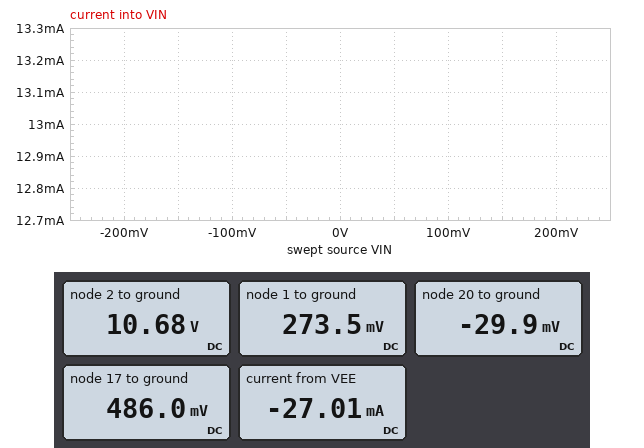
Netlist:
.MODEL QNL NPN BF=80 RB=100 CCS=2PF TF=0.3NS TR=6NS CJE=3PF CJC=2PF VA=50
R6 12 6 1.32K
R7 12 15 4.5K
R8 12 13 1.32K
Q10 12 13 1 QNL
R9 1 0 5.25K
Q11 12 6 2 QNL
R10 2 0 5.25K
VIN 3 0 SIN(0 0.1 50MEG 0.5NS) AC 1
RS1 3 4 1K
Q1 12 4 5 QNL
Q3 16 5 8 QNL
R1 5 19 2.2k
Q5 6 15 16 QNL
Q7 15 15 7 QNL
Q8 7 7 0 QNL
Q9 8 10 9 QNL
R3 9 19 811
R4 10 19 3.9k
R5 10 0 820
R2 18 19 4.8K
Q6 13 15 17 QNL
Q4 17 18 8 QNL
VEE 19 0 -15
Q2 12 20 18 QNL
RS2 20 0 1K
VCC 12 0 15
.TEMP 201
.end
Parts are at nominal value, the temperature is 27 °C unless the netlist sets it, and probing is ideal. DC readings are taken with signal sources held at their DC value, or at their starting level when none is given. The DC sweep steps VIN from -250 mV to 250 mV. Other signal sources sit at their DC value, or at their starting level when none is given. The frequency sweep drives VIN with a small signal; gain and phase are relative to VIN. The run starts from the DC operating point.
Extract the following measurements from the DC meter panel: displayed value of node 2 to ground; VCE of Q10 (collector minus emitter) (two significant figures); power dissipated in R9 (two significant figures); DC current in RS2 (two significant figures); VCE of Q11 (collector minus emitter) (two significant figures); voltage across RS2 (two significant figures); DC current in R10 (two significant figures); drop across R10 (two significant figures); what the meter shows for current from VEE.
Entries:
10.68 V
15 V
14 µW
30 µA
4.3 V
30 mV
2.0 mA
11 V
-27.01 mA
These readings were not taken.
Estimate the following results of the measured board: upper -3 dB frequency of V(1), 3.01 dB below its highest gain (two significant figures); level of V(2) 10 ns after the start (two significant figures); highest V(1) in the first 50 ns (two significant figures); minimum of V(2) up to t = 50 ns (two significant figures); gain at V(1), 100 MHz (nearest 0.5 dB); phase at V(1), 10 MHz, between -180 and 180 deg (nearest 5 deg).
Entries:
22 MHz
9.2 V
2.5 V
8.0 V
-4.5 dB
-40 deg
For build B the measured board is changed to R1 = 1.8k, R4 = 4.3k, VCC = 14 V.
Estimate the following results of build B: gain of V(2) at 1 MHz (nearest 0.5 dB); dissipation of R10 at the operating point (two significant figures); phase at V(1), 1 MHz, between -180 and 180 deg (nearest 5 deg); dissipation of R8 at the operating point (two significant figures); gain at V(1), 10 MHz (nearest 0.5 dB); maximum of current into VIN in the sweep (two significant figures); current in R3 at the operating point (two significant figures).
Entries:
33.5 dB
23 mW
10 deg
140 mW
13.5 dB
-75 µA
15 mA
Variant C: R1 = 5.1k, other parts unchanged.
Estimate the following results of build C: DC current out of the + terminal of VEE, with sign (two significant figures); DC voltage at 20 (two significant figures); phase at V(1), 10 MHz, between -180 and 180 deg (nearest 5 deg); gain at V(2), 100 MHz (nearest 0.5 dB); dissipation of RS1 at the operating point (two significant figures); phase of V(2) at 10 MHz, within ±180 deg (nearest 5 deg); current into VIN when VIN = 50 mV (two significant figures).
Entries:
-23 mA
-29 mV
-50 deg
6.5 dB
770 nW
130 deg
-28 µA
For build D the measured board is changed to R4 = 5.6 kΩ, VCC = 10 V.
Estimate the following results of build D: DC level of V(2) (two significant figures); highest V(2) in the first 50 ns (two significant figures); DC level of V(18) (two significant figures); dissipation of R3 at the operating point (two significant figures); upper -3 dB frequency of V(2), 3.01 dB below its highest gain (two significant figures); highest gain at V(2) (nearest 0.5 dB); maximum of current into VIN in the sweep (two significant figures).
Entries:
4.2 V
5.4 V
-600 mV
190 mW
43 MHz
21.5 dB
-66 µA
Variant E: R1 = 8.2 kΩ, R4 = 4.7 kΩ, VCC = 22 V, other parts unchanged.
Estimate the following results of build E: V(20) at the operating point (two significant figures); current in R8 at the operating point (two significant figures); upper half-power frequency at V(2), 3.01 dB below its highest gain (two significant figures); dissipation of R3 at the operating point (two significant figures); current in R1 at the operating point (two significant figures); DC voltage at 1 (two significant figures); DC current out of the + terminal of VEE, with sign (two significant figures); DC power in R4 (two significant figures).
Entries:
-26 mV
5.0 mA
23 MHz
180 mW
1.8 mA
15 V
-22 mA
34 mW
